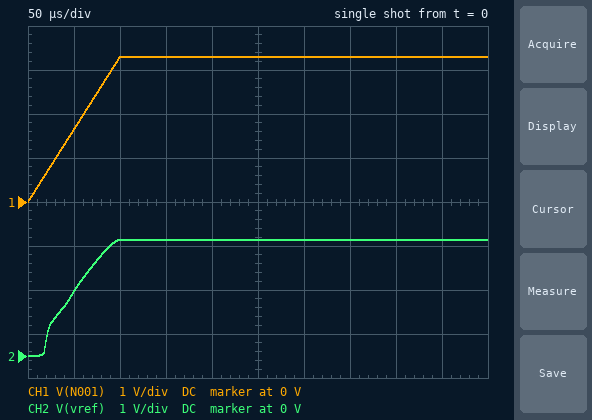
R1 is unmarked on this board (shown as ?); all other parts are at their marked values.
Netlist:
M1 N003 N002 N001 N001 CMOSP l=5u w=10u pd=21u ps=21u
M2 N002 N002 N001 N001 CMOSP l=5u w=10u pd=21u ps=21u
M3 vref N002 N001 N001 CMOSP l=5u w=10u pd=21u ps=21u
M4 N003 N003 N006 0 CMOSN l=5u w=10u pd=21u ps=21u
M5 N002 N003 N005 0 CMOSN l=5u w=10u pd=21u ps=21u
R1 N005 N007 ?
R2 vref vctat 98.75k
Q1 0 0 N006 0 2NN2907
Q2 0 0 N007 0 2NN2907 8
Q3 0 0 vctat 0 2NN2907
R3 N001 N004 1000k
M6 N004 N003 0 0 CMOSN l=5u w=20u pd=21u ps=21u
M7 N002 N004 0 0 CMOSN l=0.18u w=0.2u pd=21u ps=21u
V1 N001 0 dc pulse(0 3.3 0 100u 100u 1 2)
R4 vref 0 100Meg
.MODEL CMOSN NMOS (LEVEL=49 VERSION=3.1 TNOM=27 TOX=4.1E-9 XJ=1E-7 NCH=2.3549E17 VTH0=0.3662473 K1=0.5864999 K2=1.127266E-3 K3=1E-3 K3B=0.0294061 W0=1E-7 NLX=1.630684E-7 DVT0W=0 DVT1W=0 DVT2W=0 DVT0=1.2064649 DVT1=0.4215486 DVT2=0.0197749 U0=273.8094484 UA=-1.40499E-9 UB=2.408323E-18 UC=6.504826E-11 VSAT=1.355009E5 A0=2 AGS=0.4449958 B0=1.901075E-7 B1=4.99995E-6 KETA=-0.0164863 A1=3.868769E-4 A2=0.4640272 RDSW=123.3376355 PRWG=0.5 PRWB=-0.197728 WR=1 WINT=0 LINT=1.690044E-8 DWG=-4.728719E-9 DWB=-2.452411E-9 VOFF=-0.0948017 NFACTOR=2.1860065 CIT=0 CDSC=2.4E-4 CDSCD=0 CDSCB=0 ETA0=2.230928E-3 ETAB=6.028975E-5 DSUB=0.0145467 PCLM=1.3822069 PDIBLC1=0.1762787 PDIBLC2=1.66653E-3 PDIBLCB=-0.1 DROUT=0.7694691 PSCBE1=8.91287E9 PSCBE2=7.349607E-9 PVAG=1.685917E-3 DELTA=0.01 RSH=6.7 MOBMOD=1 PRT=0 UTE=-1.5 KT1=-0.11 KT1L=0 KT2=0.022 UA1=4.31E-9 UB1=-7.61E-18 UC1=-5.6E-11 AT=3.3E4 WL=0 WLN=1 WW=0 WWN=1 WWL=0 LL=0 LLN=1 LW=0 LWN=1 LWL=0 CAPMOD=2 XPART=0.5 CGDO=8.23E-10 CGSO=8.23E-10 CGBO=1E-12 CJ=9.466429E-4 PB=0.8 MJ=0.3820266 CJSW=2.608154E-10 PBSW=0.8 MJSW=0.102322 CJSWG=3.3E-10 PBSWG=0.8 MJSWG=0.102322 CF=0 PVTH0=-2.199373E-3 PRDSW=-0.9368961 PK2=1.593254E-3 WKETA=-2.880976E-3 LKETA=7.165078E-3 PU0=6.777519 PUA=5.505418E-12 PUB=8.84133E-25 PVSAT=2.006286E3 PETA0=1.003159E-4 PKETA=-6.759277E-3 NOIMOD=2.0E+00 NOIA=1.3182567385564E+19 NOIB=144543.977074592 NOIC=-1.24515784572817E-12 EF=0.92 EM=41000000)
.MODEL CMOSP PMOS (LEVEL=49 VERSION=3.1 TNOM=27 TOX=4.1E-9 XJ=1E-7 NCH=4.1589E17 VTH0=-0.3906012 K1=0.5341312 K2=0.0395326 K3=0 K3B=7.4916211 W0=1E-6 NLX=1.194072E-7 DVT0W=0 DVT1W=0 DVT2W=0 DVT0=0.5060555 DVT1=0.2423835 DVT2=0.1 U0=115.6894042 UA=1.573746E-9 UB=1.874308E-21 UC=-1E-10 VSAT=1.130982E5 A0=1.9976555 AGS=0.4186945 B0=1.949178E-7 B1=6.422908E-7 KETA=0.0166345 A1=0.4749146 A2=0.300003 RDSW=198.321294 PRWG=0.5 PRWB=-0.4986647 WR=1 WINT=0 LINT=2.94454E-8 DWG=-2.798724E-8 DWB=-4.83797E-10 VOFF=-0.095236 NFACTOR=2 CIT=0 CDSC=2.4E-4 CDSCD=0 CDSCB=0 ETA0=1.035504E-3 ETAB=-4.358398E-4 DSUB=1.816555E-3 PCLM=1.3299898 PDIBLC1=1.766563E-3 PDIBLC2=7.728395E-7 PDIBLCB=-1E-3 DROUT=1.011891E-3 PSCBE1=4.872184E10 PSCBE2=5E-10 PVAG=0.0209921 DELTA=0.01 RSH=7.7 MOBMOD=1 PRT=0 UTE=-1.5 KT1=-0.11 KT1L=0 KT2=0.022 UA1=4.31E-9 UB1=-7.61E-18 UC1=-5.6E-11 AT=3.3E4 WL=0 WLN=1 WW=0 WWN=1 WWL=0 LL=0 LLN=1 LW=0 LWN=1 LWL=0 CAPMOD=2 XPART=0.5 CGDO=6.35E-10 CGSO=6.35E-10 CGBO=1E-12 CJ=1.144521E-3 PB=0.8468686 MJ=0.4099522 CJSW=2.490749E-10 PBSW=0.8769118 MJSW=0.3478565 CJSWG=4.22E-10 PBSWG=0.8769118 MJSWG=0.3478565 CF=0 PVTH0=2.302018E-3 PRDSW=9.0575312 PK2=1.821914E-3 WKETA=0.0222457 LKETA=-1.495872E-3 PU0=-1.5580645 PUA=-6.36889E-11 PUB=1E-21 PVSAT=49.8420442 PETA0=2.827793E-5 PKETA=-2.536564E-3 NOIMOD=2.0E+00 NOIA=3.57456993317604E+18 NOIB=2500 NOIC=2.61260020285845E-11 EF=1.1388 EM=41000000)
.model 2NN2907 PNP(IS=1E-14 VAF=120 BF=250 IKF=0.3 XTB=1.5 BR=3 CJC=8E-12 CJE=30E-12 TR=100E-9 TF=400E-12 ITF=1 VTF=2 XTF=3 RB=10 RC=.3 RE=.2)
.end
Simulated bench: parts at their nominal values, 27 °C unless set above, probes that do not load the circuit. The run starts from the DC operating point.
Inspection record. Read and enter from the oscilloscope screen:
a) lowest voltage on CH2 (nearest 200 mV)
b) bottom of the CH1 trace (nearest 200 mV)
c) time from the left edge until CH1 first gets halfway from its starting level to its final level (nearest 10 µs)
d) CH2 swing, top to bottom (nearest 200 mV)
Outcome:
0 V
0 V
50 µs
2.6 V
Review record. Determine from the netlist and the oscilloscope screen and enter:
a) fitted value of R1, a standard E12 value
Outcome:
2.7 kΩ
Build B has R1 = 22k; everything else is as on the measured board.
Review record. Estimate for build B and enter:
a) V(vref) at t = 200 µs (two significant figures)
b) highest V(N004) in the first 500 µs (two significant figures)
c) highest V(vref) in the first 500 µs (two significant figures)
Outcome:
800 mV
410 mV
1.1 V
